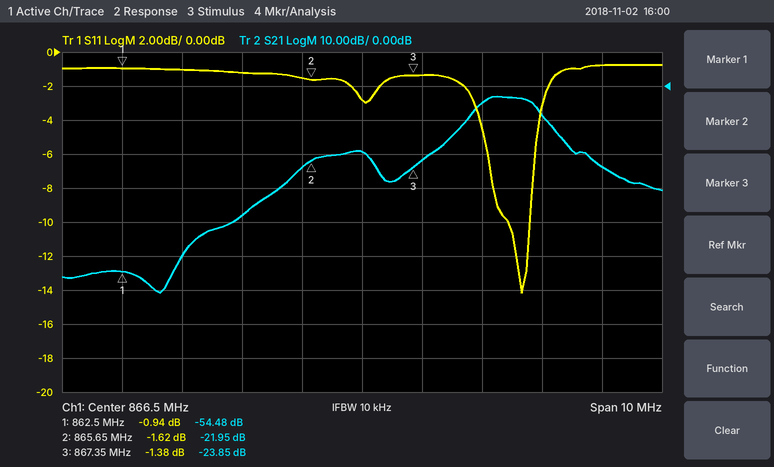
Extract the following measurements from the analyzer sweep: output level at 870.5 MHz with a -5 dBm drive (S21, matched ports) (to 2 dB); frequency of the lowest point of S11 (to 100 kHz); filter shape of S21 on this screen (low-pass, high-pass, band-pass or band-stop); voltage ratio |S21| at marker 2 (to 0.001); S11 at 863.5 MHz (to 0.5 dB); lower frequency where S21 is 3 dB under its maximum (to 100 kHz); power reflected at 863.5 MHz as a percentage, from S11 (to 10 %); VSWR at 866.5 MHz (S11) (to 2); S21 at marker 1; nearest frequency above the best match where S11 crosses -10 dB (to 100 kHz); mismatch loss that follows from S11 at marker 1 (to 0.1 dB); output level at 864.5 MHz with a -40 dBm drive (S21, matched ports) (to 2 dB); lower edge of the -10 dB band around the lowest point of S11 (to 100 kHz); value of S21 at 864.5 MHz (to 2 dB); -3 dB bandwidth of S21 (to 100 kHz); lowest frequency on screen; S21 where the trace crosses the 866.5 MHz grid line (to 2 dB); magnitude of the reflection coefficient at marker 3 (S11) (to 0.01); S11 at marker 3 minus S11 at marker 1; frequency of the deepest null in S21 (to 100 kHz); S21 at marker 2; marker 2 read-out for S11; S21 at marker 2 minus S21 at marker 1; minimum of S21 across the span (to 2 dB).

-28 dBm
869.2 MHz
band-pass
0.080
-1.0 dB
868.4 MHz
80 %
6
-54.48 dB
869.3 MHz
7.1 dB
-78 dBm
868.9 MHz
-38 dB
1.0 MHz
861.5 MHz
-20 dB
0.85
-0.44 dB
863.1 MHz
-21.95 dB
-1.62 dB
32.53 dB
-60 dB
